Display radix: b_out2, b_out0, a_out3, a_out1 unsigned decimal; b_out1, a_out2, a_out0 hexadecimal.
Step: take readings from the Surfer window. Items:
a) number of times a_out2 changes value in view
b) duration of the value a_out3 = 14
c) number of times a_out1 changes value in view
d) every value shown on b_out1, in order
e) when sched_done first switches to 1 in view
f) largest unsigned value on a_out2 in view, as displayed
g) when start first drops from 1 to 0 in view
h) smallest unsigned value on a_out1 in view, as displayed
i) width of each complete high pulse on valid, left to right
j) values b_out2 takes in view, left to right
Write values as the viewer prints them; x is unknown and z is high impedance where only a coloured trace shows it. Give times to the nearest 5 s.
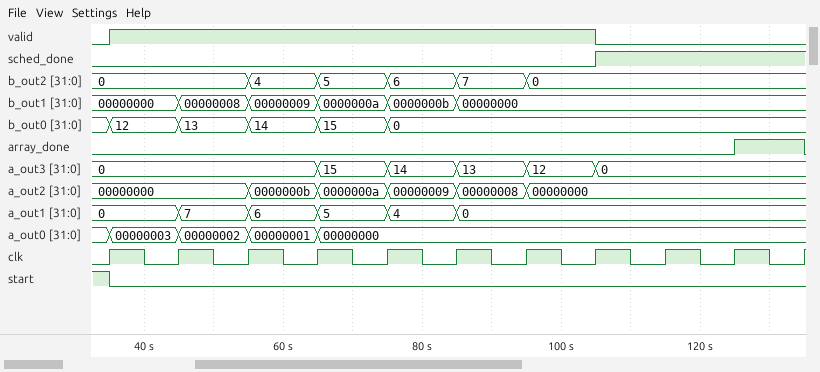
5
10 s
5
00000000, 00000008, 00000009, 0000000a, 0000000b, 00000000
105 s
0000000b
35 s
0
70 s
0, 4, 5, 6, 7, 0
